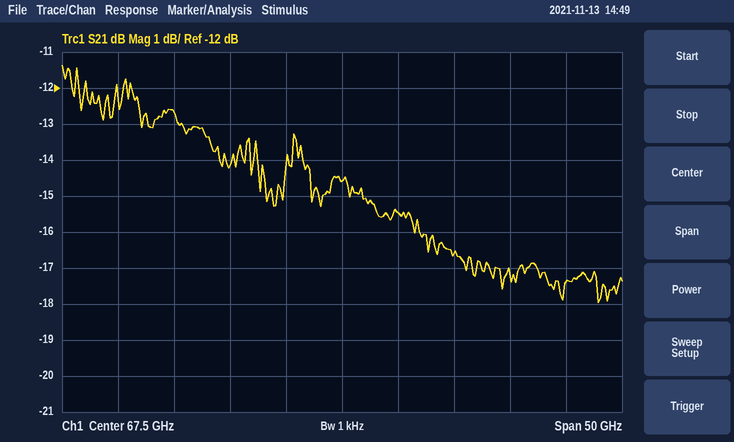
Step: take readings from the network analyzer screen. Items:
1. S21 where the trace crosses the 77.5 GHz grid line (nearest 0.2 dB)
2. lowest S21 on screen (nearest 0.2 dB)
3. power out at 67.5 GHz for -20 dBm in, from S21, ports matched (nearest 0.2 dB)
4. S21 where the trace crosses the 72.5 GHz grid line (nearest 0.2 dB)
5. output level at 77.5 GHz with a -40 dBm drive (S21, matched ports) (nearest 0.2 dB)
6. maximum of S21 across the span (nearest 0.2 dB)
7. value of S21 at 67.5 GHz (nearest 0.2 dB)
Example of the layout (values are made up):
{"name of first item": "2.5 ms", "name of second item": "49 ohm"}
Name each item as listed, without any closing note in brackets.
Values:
{"S21 where the trace crosses the 77.5 GHz grid line": "-16.6 dB", "lowest S21 on screen": "-18.0 dB", "power out at 67.5 GHz for -20 dBm in, from S21, ports matched": "-34.6 dBm", "S21 where the trace crosses the 72.5 GHz grid line": "-15.4 dB", "output level at 77.5 GHz with a -40 dBm drive (S21, matched ports)": "-56.6 dBm", "maximum of S21 across the span": "-11.4 dB", "value of S21 at 67.5 GHz": "-14.6 dB"}
